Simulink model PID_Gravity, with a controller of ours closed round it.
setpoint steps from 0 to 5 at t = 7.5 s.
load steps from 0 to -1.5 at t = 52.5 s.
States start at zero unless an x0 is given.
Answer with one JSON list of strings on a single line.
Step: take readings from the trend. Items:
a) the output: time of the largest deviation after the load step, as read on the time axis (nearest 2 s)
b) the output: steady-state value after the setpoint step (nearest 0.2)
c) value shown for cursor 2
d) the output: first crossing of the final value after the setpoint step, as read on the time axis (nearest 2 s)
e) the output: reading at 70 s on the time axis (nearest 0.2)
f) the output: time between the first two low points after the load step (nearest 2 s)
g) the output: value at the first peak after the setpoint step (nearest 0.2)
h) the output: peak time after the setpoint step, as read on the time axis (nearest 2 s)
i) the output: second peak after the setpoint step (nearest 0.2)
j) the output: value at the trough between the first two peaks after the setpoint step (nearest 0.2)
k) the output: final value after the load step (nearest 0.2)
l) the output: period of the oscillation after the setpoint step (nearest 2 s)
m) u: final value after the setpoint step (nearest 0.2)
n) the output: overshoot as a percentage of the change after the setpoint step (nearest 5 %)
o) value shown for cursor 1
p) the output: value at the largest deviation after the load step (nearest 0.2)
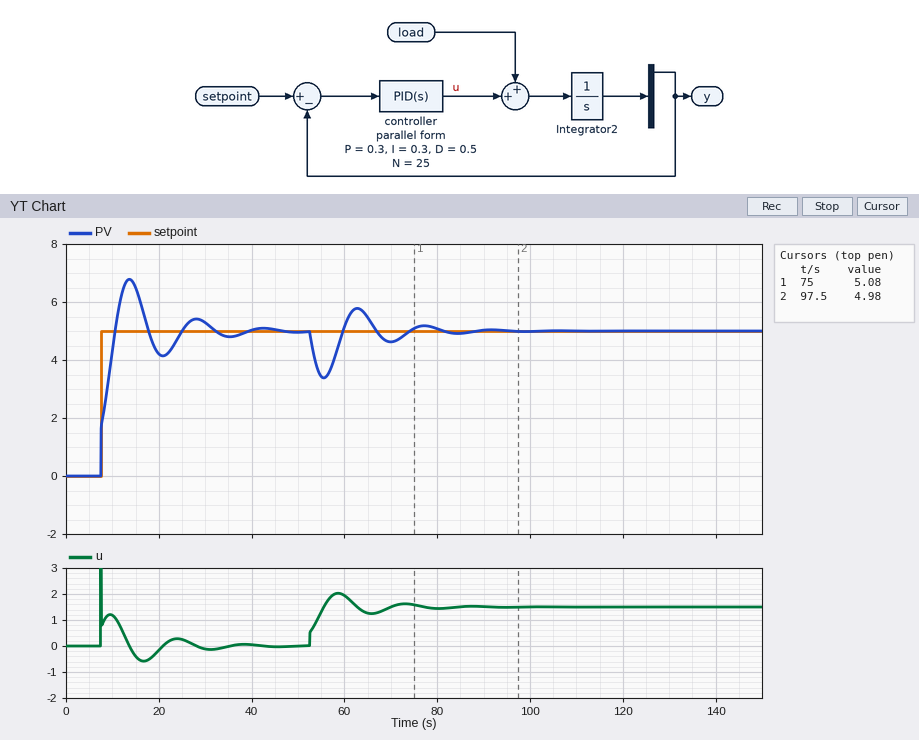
["56 s", "5.0", "4.98", "10 s", "4.6", "14 s", "6.8", "14 s", "5.4", "4.2", "5.0", "14 s", "0.0", "35 %", "5.08", "3.4"]
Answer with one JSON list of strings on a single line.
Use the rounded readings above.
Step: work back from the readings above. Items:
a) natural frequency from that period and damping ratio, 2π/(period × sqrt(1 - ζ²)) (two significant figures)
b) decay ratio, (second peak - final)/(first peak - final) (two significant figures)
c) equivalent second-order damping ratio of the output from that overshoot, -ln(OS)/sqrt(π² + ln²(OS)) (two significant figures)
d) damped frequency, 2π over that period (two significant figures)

["0.47 rad/s", "0.22", "0.32", "0.45 rad/s"]
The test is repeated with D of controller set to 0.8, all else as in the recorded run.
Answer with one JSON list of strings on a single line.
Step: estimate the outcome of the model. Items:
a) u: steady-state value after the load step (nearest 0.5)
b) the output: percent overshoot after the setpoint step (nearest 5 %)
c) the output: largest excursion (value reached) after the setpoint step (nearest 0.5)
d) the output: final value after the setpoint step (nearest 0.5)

["1.5", "30 %", "6.5", "5.0"]
